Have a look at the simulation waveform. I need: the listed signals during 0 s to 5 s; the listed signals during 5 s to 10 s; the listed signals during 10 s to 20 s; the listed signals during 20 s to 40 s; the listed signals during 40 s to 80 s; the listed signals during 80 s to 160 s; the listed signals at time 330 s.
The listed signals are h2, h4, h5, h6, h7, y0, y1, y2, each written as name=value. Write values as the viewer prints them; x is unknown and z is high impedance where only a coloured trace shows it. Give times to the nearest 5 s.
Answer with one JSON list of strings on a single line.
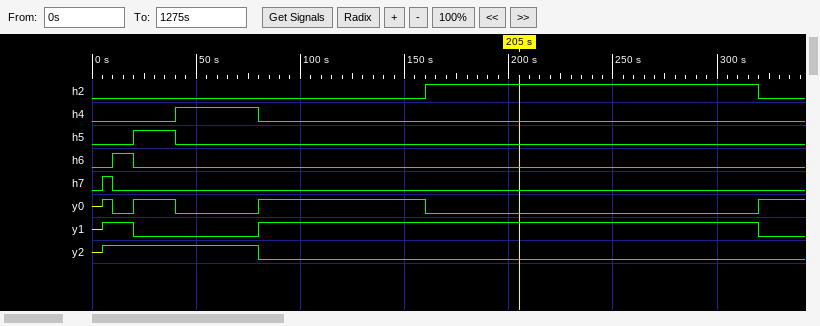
["h2=0, h4=0, h5=0, h6=0, h7=0, y0=z, y1=z, y2=z", "h2=0, h4=0, h5=0, h6=0, h7=1, y0=1, y1=1, y2=1", "h2=0, h4=0, h5=0, h6=1, h7=0, y0=0, y1=1, y2=1", "h2=0, h4=0, h5=1, h6=0, h7=0, y0=1, y1=0, y2=1", "h2=0, h4=1, h5=0, h6=0, h7=0, y0=0, y1=0, y2=1", "h2=0, h4=0, h5=0, h6=0, h7=0, y0=1, y1=1, y2=0", "h2=0, h4=0, h5=0, h6=0, h7=0, y0=1, y1=0, y2=0"]
